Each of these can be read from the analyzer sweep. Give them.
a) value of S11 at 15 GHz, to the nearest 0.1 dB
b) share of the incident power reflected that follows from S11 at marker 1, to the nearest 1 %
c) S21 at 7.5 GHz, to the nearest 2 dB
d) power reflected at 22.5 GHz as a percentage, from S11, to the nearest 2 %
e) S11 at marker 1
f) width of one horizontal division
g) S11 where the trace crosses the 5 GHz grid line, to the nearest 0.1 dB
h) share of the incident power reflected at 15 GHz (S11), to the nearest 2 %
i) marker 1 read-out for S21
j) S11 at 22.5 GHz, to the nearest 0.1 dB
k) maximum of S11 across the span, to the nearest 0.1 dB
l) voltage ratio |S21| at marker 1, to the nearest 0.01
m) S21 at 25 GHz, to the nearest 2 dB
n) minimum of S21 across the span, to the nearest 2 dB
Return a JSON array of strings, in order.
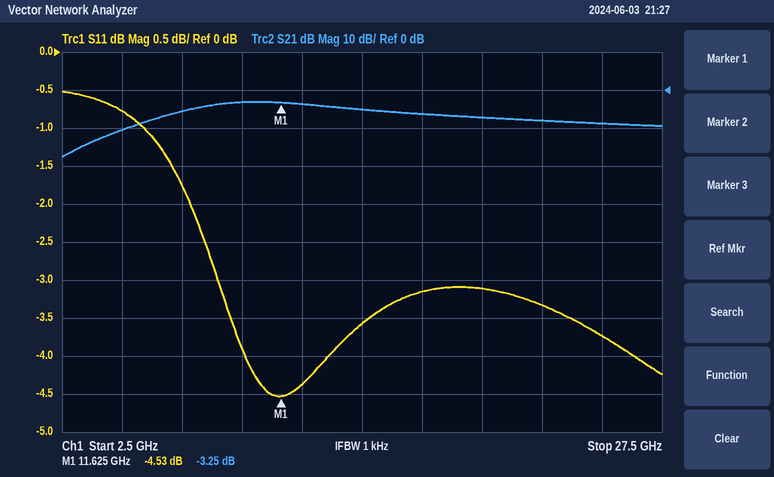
["-3.6 dB", "35 %", "-6 dB", "46 %", "-4.53 dB", "2.5 GHz", "-0.8 dB", "44 %", "-3.25 dB", "-3.3 dB", "-0.5 dB", "0.69", "-8 dB", "-18 dB"]
